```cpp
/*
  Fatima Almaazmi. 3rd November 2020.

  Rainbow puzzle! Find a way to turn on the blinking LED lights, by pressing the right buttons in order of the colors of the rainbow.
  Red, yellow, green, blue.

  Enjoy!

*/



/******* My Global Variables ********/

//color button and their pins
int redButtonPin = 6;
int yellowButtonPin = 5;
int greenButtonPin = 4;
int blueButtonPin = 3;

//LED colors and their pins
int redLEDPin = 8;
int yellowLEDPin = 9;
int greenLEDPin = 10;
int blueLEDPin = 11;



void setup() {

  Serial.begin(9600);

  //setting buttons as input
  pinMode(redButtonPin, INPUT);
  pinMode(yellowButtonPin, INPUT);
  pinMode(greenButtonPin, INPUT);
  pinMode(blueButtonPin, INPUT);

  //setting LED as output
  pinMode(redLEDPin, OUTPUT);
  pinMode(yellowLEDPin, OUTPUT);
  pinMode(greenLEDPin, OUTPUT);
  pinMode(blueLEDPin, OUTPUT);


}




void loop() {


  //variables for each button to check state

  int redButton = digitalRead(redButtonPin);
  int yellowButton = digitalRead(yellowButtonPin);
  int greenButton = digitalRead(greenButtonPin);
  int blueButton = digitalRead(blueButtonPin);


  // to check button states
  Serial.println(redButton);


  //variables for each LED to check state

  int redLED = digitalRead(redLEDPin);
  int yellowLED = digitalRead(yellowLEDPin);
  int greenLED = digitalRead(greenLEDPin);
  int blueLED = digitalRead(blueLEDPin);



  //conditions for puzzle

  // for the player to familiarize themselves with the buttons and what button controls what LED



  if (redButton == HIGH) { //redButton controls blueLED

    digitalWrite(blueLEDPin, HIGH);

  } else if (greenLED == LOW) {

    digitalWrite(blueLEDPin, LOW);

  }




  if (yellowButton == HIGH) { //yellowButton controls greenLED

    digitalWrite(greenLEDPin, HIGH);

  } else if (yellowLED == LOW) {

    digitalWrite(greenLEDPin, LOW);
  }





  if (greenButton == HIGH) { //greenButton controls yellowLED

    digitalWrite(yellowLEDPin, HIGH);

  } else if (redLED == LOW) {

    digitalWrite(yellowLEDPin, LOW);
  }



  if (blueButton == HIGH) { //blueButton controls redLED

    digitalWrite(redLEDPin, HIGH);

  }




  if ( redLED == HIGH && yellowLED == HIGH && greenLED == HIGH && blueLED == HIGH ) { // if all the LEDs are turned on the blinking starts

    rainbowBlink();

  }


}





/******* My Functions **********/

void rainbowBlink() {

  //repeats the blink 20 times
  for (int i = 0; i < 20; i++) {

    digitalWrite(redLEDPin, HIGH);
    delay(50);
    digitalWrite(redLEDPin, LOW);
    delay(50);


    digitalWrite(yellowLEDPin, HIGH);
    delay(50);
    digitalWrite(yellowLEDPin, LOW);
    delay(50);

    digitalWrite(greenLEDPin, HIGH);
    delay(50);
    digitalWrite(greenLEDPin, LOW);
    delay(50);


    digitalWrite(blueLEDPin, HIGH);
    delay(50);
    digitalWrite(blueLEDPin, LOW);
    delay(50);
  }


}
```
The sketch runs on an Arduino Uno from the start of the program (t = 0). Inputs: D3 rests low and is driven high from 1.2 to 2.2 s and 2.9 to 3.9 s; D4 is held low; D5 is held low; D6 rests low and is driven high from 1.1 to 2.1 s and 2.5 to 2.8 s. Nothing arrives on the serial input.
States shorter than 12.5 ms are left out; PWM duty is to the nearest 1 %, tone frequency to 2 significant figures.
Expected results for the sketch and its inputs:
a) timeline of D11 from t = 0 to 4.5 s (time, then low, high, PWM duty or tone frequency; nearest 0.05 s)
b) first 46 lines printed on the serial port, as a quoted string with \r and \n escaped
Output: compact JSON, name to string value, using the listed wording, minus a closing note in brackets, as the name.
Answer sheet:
{"timeline of D11 from t = 0 to 4.5 s": "0 s low; 1.1 s high; 2.1 s low; 2.5 s high; 2.8 s low", "first 46 lines printed on the serial port, as a quoted string with \\r and \\n escaped": "\"0\\r\\n0\\r\\n0\\r\\n0\\r\\n0\\r\\n0\\r\\n0\\r\\n0\\r\\n0\\r\\n0\\r\\n0\\r\\n0\\r\\n0\\r\\n0\\r\\n0\\r\\n0\\r\\n0\\r\\n0\\r\\n0\\r\\n0\\r\\n0\\r\\n0\\r\\n0\\r\\n0\\r\\n0\\r\\n0\\r\\n0\\r\\n0\\r\\n0\\r\\n0\\r\\n0\\r\\n0\\r\\n0\\r\\n0\\r\\n0\\r\\n0\\r\\n0\\r\\n0\\r\\n0\\r\\n0\\r\\n0\\r\\n0\\r\\n0\\r\\n0\\r\\n0\\r\\n0\\r\\n\""}
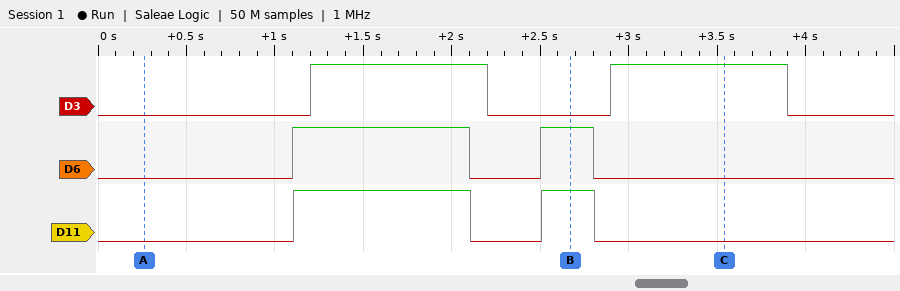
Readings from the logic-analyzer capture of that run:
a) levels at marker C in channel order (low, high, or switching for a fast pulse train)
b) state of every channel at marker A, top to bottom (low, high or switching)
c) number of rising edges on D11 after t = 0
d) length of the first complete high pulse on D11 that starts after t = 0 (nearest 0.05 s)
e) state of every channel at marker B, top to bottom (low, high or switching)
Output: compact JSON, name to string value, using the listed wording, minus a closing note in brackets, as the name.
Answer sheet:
{"levels at marker C in channel order": "D3 high, D6 low, D11 low", "state of every channel at marker A, top to bottom": "D3 low, D6 low, D11 low", "number of rising edges on D11 after t = 0": "2", "length of the first complete high pulse on D11 that starts after t = 0": "1.00 s", "state of every channel at marker B, top to bottom": "D3 low, D6 high, D11 high"}
